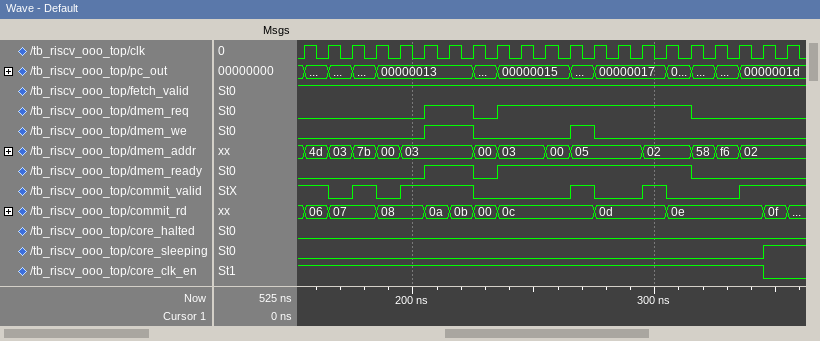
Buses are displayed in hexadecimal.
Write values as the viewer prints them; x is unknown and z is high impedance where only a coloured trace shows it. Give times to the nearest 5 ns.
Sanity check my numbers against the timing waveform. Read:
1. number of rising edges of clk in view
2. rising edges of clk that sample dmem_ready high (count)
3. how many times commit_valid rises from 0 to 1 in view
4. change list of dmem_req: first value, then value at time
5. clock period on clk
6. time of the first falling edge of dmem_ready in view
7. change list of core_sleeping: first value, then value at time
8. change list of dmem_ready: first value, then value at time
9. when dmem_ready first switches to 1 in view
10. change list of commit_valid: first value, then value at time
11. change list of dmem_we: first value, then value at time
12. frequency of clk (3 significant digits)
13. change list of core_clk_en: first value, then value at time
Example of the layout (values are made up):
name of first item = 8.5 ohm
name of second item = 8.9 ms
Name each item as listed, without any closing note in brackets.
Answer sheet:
number of rising edges of clk in view = 21
rising edges of clk that sample dmem_ready high = 10
how many times commit_valid rises from 0 to 1 in view = 5
change list of dmem_req: first value, then value at time = 0, 1 at 205 ns, 0 at 225 ns, 1 at 235 ns, 0 at 315 ns
clock period on clk = 10 ns
time of the first falling edge of dmem_ready in view = 225 ns
change list of core_sleeping: first value, then value at time = 0, 1 at 345 ns
change list of dmem_ready: first value, then value at time = 0, 1 at 205 ns, 0 at 225 ns, 1 at 235 ns, 0 at 315 ns
when dmem_ready first switches to 1 in view = 205 ns
change list of commit_valid: first value, then value at time = 1, 0 at 165 ns, 1 at 175 ns, 0 at 185 ns, 1 at 195 ns, 0 at 225 ns, 1 at 265 ns, 0 at 275 ns, 1 at 295 ns, 0 at 305 ns, 1 at 335 ns
change list of dmem_we: first value, then value at time = 0, 1 at 205 ns, 0 at 225 ns, 1 at 265 ns, 0 at 275 ns
frequency of clk = 100 MHz
change list of core_clk_en: first value, then value at time = 1, 0 at 345 ns
